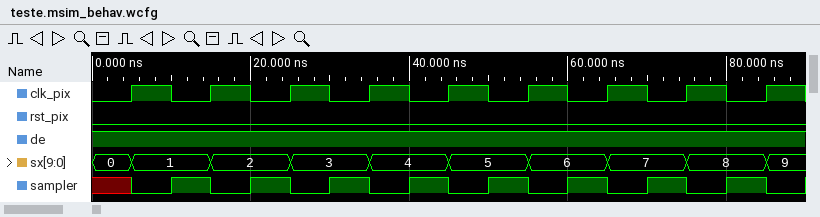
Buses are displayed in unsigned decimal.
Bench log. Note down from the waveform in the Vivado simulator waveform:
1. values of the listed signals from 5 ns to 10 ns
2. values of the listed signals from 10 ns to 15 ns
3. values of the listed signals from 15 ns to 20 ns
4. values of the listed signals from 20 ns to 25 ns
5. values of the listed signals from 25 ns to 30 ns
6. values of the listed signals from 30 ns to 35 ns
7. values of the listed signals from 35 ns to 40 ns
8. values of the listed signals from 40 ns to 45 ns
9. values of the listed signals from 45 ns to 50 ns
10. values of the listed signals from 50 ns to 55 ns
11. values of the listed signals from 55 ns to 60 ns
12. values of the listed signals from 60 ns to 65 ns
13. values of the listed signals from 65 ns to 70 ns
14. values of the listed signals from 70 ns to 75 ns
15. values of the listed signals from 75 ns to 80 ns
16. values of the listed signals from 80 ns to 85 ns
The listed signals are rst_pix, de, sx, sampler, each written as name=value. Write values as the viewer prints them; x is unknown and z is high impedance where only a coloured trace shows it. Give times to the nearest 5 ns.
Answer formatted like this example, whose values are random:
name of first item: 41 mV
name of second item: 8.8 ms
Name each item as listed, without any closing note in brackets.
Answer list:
values of the listed signals from 5 ns to 10 ns: rst_pix=0, de=1, sx=1, sampler=0
values of the listed signals from 10 ns to 15 ns: rst_pix=0, de=1, sx=1, sampler=1
values of the listed signals from 15 ns to 20 ns: rst_pix=0, de=1, sx=2, sampler=0
values of the listed signals from 20 ns to 25 ns: rst_pix=0, de=1, sx=2, sampler=1
values of the listed signals from 25 ns to 30 ns: rst_pix=0, de=1, sx=3, sampler=0
values of the listed signals from 30 ns to 35 ns: rst_pix=0, de=1, sx=3, sampler=1
values of the listed signals from 35 ns to 40 ns: rst_pix=0, de=1, sx=4, sampler=0
values of the listed signals from 40 ns to 45 ns: rst_pix=0, de=1, sx=4, sampler=1
values of the listed signals from 45 ns to 50 ns: rst_pix=0, de=1, sx=5, sampler=0
values of the listed signals from 50 ns to 55 ns: rst_pix=0, de=1, sx=5, sampler=1
values of the listed signals from 55 ns to 60 ns: rst_pix=0, de=1, sx=6, sampler=0
values of the listed signals from 60 ns to 65 ns: rst_pix=0, de=1, sx=6, sampler=1
values of the listed signals from 65 ns to 70 ns: rst_pix=0, de=1, sx=7, sampler=0
values of the listed signals from 70 ns to 75 ns: rst_pix=0, de=1, sx=7, sampler=1
values of the listed signals from 75 ns to 80 ns: rst_pix=0, de=1, sx=8, sampler=0
values of the listed signals from 80 ns to 85 ns: rst_pix=0, de=1, sx=8, sampler=1
